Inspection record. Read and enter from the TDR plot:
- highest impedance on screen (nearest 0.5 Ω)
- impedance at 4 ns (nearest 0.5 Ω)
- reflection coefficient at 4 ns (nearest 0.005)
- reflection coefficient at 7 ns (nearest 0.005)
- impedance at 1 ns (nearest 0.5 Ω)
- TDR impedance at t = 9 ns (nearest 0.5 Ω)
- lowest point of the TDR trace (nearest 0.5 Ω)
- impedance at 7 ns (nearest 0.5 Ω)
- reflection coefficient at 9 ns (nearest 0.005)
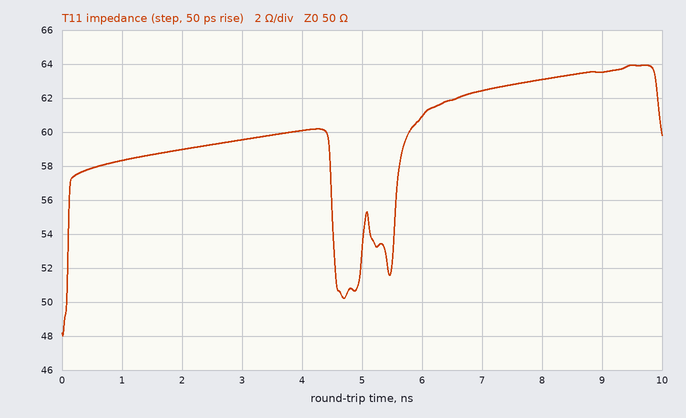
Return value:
64.0 Ω
60.0 Ω
+0.090
+0.110
58.5 Ω
63.5 Ω
48.0 Ω
62.5 Ω
+0.120
